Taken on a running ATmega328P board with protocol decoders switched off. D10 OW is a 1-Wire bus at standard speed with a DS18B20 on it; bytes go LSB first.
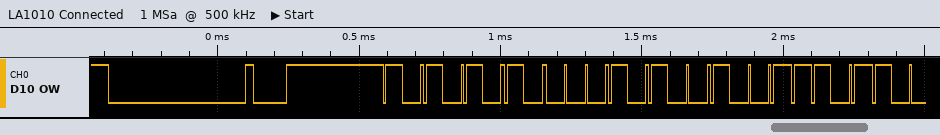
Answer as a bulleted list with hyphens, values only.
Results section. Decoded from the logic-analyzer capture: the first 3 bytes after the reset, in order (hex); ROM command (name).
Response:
- 55 28 B9
- Match ROM
